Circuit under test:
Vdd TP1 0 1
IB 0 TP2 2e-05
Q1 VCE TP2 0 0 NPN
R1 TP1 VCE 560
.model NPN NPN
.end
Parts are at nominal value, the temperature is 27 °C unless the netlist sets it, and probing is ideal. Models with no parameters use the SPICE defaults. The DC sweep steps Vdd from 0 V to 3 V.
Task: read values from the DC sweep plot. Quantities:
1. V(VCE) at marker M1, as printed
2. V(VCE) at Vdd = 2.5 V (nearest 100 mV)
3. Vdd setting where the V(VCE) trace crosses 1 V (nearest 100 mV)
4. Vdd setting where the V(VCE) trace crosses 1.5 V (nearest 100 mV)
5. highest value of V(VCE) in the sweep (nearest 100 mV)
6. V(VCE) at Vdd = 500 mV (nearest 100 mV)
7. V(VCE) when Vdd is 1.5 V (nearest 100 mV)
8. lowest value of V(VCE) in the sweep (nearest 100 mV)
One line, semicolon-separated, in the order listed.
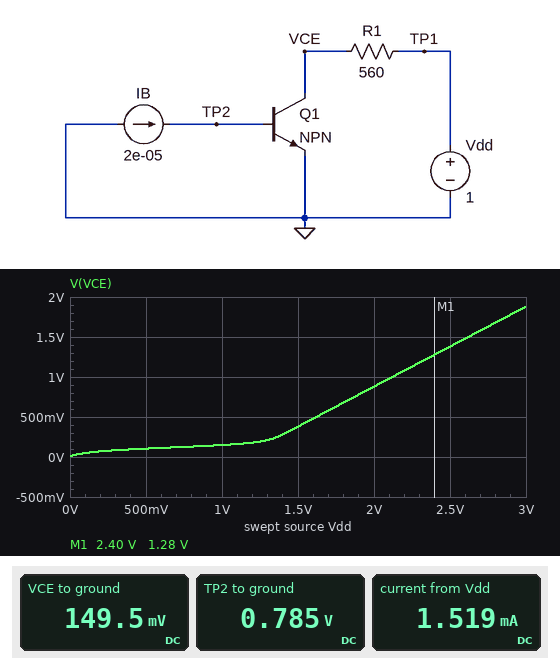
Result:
1.28 V; 1.4 V; 2.1 V; 2.6 V; 1.9 V; 100 mV; 400 mV; 0 V
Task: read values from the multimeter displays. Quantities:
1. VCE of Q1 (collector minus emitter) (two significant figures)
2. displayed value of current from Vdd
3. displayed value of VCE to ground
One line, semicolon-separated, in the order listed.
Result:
150 mV; 1.519 mA; 149.5 mV
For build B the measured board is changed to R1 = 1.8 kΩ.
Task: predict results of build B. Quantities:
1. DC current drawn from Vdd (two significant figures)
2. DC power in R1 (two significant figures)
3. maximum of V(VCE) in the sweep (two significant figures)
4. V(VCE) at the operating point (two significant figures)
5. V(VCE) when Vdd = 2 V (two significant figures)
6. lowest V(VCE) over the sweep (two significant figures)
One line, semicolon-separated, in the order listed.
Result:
500 µA; 460 µW; 150 mV; 93 mV; 120 mV; 13 mV
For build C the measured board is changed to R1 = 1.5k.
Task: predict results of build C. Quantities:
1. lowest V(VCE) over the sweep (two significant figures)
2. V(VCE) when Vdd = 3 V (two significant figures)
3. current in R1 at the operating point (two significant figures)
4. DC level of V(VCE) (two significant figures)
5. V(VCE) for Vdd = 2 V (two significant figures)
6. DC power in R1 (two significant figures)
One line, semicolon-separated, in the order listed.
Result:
12 mV; 190 mV; 600 µA; 99 mV; 130 mV; 540 µW
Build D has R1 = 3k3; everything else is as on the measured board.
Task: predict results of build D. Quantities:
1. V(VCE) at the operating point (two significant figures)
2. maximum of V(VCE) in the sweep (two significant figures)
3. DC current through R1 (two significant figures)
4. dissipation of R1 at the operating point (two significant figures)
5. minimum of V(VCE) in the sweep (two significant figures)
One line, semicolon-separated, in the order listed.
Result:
76 mV; 110 mV; 280 µA; 260 µW; 15 mV
